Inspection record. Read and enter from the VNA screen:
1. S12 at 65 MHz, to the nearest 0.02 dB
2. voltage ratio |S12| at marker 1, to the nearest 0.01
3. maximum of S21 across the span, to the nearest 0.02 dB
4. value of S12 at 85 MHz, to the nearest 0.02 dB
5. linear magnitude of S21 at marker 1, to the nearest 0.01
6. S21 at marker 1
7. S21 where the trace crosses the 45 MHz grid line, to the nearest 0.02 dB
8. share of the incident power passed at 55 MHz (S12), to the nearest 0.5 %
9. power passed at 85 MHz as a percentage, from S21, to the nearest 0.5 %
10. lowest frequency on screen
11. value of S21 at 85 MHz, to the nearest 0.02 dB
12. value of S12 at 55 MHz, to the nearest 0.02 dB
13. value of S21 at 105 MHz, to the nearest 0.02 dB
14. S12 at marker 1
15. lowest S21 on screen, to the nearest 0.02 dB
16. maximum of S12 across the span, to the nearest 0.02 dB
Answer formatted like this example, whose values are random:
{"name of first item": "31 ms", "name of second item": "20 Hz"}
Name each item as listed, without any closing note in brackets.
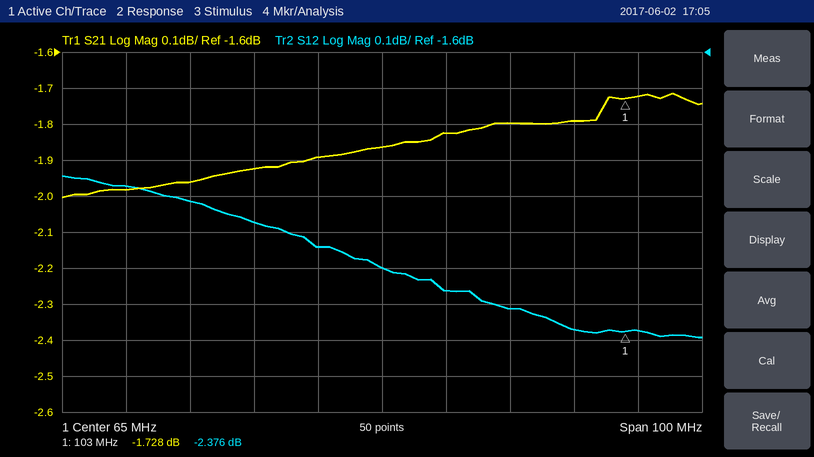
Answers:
{"S12 at 65 MHz, to the nearest 0.02 dB": "-2.20 dB", "voltage ratio |S12| at marker 1, to the nearest 0.01": "0.76", "maximum of S21 across the span, to the nearest 0.02 dB": "-1.72 dB", "value of S12 at 85 MHz, to the nearest 0.02 dB": "-2.32 dB", "linear magnitude of S21 at marker 1, to the nearest 0.01": "0.82", "S21 at marker 1": "-1.728 dB", "S21 where the trace crosses the 45 MHz grid line, to the nearest 0.02 dB": "-1.92 dB", "share of the incident power passed at 55 MHz (S12), to the nearest 0.5 %": "61.0 %", "power passed at 85 MHz as a percentage, from S21, to the nearest 0.5 %": "66.0 %", "lowest frequency on screen": "15 MHz", "value of S21 at 85 MHz, to the nearest 0.02 dB": "-1.80 dB", "value of S12 at 55 MHz, to the nearest 0.02 dB": "-2.14 dB", "value of S21 at 105 MHz, to the nearest 0.02 dB": "-1.72 dB", "S12 at marker 1": "-2.376 dB", "lowest S21 on screen, to the nearest 0.02 dB": "-2.00 dB", "maximum of S12 across the span, to the nearest 0.02 dB": "-1.94 dB"}
